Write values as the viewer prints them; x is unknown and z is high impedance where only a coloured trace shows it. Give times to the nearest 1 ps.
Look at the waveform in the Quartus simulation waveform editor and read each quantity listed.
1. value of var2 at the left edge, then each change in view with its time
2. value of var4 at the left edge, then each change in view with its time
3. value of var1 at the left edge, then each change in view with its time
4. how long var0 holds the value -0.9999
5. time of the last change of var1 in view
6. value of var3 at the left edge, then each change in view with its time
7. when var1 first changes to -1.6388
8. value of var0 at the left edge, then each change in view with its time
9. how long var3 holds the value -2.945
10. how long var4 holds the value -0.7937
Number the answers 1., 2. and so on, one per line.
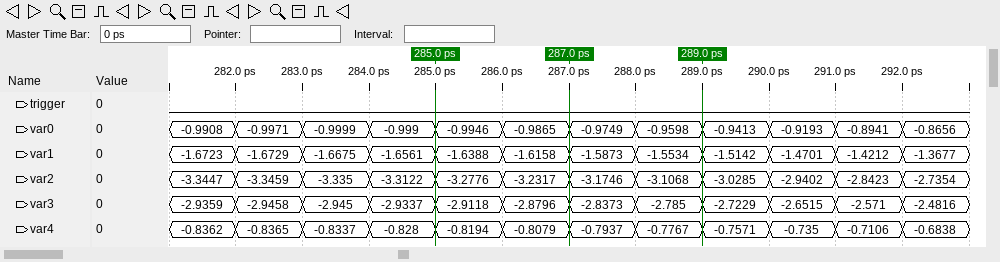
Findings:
1. -3.3447, -3.3459 at 282 ps, -3.335 at 283 ps, -3.3122 at 284 ps, -3.2776 at 285 ps, -3.2317 at 286 ps, -3.1746 at 287 ps, -3.1068 at 288 ps, -3.0285 at 289 ps, -2.9402 at 290 ps, -2.8423 at 291 ps, -2.7354 at 292 ps
2. -0.8362, -0.8365 at 282 ps, -0.8337 at 283 ps, -0.828 at 284 ps, -0.8194 at 285 ps, -0.8079 at 286 ps, -0.7937 at 287 ps, -0.7767 at 288 ps, -0.7571 at 289 ps, -0.735 at 290 ps, -0.7106 at 291 ps, -0.6838 at 292 ps
3. -1.6723, -1.6729 at 282 ps, -1.6675 at 283 ps, -1.6561 at 284 ps, -1.6388 at 285 ps, -1.6158 at 286 ps, -1.5873 at 287 ps, -1.5534 at 288 ps, -1.5142 at 289 ps, -1.4701 at 290 ps, -1.4212 at 291 ps, -1.3677 at 292 ps
4. 1 ps
5. 292 ps
6. -2.9359, -2.9458 at 282 ps, -2.945 at 283 ps, -2.9337 at 284 ps, -2.9118 at 285 ps, -2.8796 at 286 ps, -2.8373 at 287 ps, -2.785 at 288 ps, -2.7229 at 289 ps, -2.6515 at 290 ps, -2.571 at 291 ps, -2.4816 at 292 ps
7. 285 ps
8. -0.9908, -0.9971 at 282 ps, -0.9999 at 283 ps, -0.999 at 284 ps, -0.9946 at 285 ps, -0.9865 at 286 ps, -0.9749 at 287 ps, -0.9598 at 288 ps, -0.9413 at 289 ps, -0.9193 at 290 ps, -0.8941 at 291 ps, -0.8656 at 292 ps
9. 1 ps
10. 1 ps
